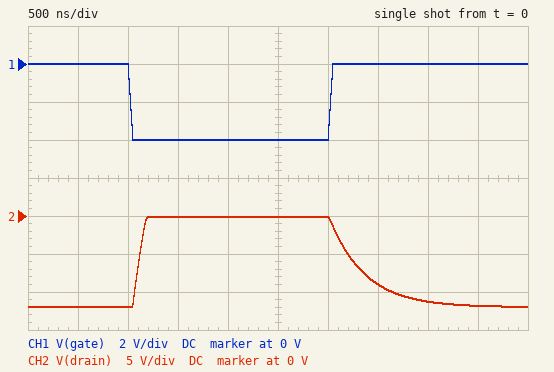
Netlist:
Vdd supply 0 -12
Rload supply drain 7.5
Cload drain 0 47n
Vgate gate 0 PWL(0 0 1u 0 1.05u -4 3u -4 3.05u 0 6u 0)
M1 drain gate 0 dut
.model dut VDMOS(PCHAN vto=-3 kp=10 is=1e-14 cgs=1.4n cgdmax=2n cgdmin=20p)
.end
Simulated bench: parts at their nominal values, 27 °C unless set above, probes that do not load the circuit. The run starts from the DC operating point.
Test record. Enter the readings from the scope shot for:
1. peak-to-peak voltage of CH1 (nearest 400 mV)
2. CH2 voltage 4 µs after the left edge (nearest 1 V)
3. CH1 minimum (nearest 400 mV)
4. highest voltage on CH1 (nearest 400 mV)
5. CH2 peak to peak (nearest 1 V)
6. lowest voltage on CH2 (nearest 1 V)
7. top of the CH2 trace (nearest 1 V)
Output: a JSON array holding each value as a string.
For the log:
["4.0 V", "-11 V", "-4.0 V", "0 V", "12 V", "-12 V", "0 V"]
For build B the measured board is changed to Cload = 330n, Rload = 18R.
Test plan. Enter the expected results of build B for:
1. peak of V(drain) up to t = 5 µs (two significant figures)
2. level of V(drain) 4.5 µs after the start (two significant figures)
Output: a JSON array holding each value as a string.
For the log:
["-68 mV", "-2.7 V"]
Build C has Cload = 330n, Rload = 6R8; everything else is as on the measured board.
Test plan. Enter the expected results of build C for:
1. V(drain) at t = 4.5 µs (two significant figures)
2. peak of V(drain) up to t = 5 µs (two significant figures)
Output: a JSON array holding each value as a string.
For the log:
["-5.9 V", "-190 mV"]
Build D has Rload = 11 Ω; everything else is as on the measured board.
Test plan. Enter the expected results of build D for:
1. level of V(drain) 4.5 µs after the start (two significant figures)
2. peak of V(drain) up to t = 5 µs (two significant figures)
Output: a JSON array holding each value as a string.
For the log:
["-11 V", "-110 mV"]
